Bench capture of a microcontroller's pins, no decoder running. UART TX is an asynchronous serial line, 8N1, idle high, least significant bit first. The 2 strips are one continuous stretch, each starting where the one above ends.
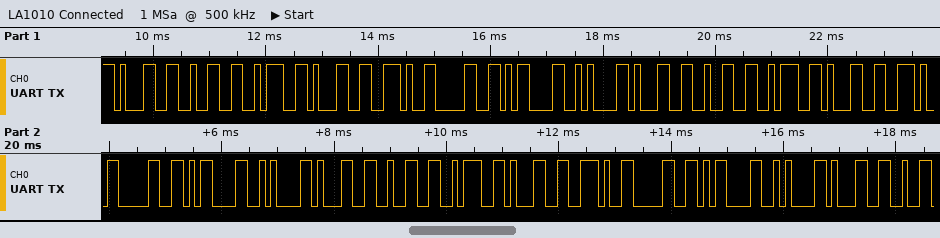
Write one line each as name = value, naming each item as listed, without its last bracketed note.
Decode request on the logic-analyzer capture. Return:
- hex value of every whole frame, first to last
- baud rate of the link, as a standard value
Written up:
hex value of every whole frame, first to last = 31 32 3A 31 2E 30 0D 0A 31 32 3A 31 2E 30 0D 0A 31 32 3A 31 2E 30 0D 0A 31
baud rate of the link, as a standard value = 9600 baud
